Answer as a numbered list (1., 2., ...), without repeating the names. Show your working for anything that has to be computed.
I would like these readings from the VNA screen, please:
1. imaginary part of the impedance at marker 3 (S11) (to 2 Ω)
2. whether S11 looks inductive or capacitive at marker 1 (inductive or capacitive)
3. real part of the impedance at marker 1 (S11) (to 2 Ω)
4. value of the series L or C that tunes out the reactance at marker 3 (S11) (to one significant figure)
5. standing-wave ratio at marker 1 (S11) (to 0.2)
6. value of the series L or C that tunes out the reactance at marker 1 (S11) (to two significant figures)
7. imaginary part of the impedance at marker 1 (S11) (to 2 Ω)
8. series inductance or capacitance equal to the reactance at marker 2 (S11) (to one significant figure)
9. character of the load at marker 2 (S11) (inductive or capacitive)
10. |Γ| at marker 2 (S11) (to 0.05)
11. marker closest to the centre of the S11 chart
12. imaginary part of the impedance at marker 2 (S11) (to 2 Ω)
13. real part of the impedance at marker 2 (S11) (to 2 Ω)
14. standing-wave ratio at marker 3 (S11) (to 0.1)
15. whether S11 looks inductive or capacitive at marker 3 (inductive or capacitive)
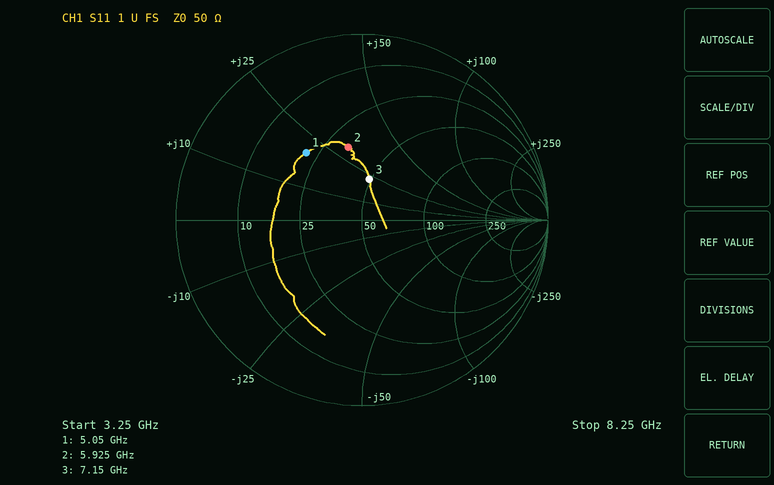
1. +22 Ω
2. inductive
3. 22 Ω
4. C = 1/(2π × 7.15 GHz × 22 Ω) ≈ 1.0 pF
5. 2.8
6. C = 1/(2π × 5.05 GHz × 20 Ω) ≈ 1.6 pF
7. +20 Ω
8. L = 30 Ω/(2π × 5.925 GHz) ≈ 806 pH, so 800 pH to one significant figure
9. inductive
10. 0.40
11. marker 3
12. +30 Ω
13. 32 Ω
14. 1.6
15. inductive
